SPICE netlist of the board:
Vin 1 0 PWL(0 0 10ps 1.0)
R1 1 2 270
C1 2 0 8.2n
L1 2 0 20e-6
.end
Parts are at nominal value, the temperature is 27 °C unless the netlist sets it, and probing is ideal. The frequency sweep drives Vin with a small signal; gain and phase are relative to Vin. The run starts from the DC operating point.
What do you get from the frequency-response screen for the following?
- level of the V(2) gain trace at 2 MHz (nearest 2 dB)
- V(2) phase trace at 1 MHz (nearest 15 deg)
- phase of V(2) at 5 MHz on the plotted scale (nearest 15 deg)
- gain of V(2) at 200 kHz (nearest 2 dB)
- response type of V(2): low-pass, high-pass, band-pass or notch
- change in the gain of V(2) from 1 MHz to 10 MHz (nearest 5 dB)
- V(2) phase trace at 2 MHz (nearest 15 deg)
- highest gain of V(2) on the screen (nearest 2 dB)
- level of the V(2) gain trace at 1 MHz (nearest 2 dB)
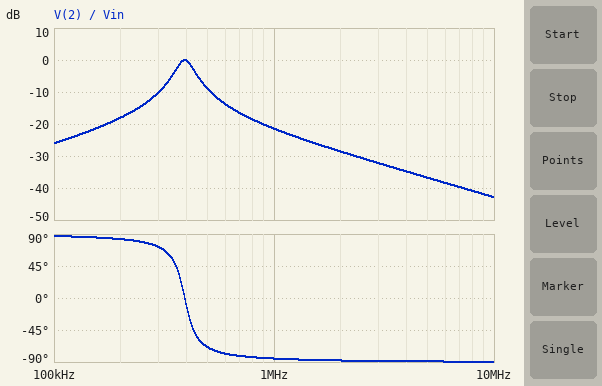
-28 dB
-90 deg
-90 deg
-18 dB
band-pass
-20 dB
-90 deg
0 dB
-22 dB
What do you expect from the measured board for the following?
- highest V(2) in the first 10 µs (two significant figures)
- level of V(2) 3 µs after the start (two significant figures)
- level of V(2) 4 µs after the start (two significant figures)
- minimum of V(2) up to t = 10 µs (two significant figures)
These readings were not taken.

160 mV
83 mV
-30 mV
-120 mV
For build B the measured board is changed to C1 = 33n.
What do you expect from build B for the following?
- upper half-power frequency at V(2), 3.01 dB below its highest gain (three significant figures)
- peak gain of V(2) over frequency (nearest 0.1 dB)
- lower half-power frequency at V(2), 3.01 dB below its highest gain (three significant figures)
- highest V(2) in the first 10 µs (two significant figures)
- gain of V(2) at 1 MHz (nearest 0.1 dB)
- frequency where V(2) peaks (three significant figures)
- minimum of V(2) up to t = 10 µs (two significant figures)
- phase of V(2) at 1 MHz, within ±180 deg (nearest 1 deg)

205 kHz
0 dB
187 kHz
85 mV
-34.6 dB
196 kHz
-74 mV
-89 deg
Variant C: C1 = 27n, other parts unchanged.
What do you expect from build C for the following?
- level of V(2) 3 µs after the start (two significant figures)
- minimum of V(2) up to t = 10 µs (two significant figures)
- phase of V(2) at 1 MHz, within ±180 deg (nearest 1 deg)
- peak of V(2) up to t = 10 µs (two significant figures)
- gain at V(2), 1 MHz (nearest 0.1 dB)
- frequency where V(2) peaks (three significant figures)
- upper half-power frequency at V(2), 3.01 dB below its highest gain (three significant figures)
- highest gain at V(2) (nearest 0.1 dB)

-66 mV
-80 mV
-89 deg
93 mV
-32.8 dB
217 kHz
228 kHz
0 dB
